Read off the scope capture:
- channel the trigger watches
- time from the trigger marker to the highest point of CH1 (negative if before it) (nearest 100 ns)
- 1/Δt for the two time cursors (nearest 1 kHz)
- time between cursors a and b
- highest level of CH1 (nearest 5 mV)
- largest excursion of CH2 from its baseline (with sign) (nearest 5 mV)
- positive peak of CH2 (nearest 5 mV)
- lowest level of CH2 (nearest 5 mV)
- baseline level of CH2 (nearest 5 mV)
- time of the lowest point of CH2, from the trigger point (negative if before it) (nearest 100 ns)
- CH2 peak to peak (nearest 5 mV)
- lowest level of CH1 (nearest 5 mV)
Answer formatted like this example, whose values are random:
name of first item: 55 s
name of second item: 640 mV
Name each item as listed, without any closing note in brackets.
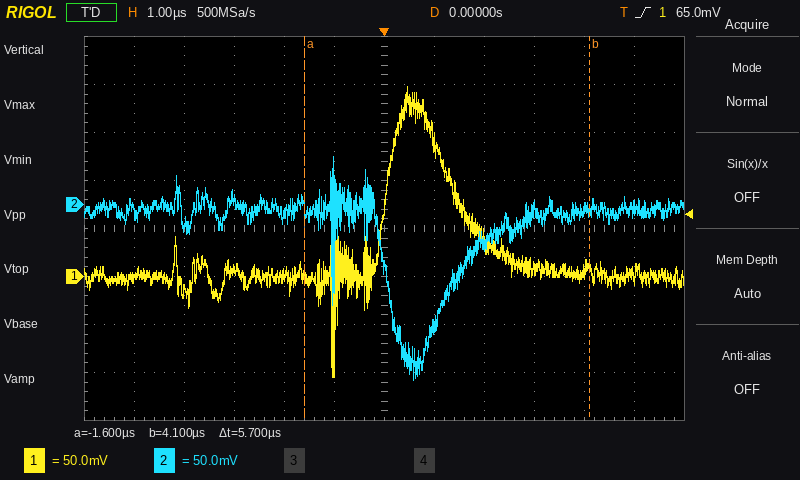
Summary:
channel the trigger watches: CH1
time from the trigger marker to the highest point of CH1 (negative if before it): +500 ns
1/Δt for the two time cursors: 175 kHz
time between cursors a and b: 5.7 µs
highest level of CH1: 200 mV
largest excursion of CH2 from its baseline (with sign): -175 mV
positive peak of CH2: 50 mV
lowest level of CH2: -180 mV
baseline level of CH2: -5 mV
time of the lowest point of CH2, from the trigger point (negative if before it): +600 ns
CH2 peak to peak: 230 mV
lowest level of CH1: -105 mV
